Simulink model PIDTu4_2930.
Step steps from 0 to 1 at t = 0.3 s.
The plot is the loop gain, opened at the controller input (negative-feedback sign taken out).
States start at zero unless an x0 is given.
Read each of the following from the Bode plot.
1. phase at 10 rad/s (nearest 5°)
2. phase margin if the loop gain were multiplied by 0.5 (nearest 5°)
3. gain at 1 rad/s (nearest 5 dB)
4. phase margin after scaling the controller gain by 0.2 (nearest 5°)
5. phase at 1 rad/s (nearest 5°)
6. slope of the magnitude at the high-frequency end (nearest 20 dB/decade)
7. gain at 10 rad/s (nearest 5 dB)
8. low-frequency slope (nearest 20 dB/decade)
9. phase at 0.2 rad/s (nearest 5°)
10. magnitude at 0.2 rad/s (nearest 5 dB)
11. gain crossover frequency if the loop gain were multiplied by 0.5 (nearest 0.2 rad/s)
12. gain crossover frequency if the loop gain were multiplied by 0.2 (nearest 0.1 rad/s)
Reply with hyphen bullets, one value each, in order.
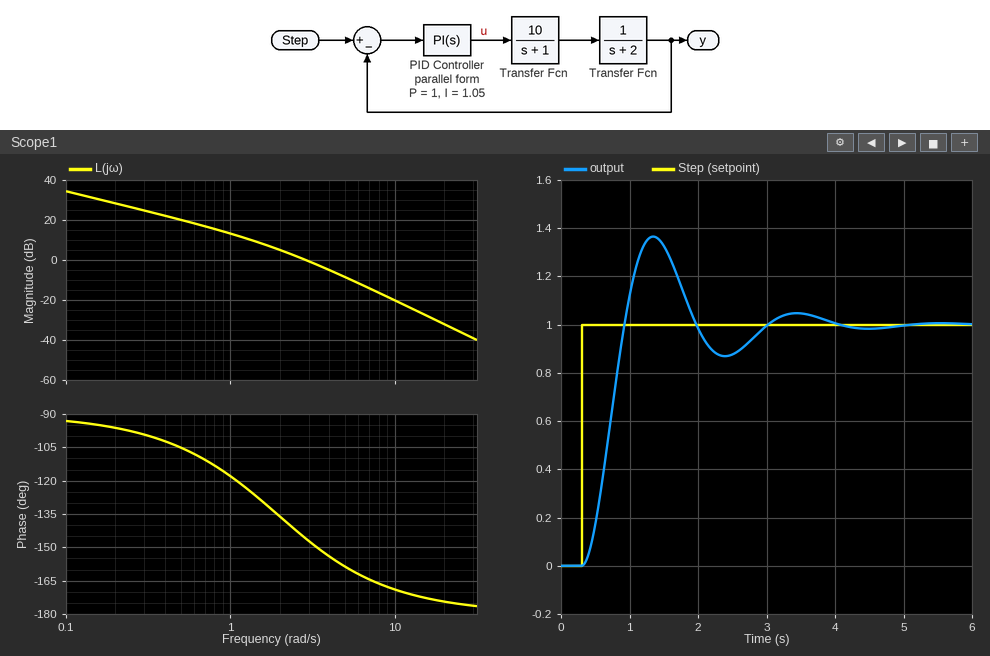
- -170°
- 45°
- 15 dB
- 65°
- -120°
- -40 dB/decade
- -20 dB
- -20 dB/decade
- -95°
- 30 dB
- 1.8 rad/s
- 0.9 rad/s
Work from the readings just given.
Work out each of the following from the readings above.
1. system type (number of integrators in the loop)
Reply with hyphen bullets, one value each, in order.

- 1
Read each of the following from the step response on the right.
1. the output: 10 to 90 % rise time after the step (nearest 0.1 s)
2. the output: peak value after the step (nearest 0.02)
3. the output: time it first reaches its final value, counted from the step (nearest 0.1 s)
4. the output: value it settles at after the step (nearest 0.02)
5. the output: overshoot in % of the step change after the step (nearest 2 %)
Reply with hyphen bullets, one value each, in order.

- 0.4 s
- 1.36
- 0.6 s
- 1.00
- 36 %
